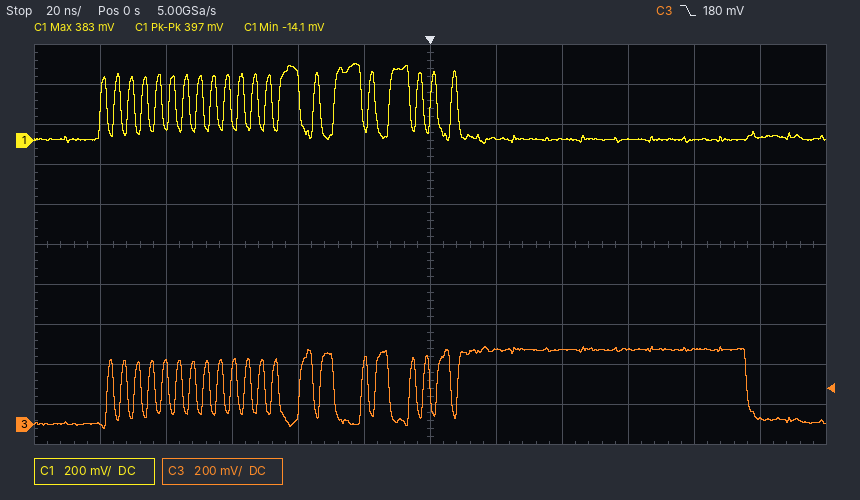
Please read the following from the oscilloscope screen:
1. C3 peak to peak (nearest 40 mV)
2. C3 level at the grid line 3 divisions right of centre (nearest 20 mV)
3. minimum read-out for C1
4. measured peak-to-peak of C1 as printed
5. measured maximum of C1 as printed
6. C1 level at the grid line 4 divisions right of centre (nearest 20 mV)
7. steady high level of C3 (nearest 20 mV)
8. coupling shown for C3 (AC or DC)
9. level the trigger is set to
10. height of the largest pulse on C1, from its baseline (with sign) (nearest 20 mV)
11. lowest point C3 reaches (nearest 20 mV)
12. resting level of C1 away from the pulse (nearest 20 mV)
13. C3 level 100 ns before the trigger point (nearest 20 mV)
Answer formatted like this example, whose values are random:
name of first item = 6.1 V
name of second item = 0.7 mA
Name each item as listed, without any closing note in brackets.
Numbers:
C3 peak to peak = 400 mV
C3 level at the grid line 3 divisions right of centre = 380 mV
minimum read-out for C1 = -14.1 mV
measured peak-to-peak of C1 as printed = 397 mV
measured maximum of C1 as printed = 383 mV
C1 level at the grid line 4 divisions right of centre = 0 mV
steady high level of C3 = 380 mV
coupling shown for C3 = DC
level the trigger is set to = 180 mV
height of the largest pulse on C1, from its baseline (with sign) = +380 mV
lowest point C3 reaches = -20 mV
resting level of C1 away from the pulse = 0 mV
C3 level 100 ns before the trigger point = 0 mV
